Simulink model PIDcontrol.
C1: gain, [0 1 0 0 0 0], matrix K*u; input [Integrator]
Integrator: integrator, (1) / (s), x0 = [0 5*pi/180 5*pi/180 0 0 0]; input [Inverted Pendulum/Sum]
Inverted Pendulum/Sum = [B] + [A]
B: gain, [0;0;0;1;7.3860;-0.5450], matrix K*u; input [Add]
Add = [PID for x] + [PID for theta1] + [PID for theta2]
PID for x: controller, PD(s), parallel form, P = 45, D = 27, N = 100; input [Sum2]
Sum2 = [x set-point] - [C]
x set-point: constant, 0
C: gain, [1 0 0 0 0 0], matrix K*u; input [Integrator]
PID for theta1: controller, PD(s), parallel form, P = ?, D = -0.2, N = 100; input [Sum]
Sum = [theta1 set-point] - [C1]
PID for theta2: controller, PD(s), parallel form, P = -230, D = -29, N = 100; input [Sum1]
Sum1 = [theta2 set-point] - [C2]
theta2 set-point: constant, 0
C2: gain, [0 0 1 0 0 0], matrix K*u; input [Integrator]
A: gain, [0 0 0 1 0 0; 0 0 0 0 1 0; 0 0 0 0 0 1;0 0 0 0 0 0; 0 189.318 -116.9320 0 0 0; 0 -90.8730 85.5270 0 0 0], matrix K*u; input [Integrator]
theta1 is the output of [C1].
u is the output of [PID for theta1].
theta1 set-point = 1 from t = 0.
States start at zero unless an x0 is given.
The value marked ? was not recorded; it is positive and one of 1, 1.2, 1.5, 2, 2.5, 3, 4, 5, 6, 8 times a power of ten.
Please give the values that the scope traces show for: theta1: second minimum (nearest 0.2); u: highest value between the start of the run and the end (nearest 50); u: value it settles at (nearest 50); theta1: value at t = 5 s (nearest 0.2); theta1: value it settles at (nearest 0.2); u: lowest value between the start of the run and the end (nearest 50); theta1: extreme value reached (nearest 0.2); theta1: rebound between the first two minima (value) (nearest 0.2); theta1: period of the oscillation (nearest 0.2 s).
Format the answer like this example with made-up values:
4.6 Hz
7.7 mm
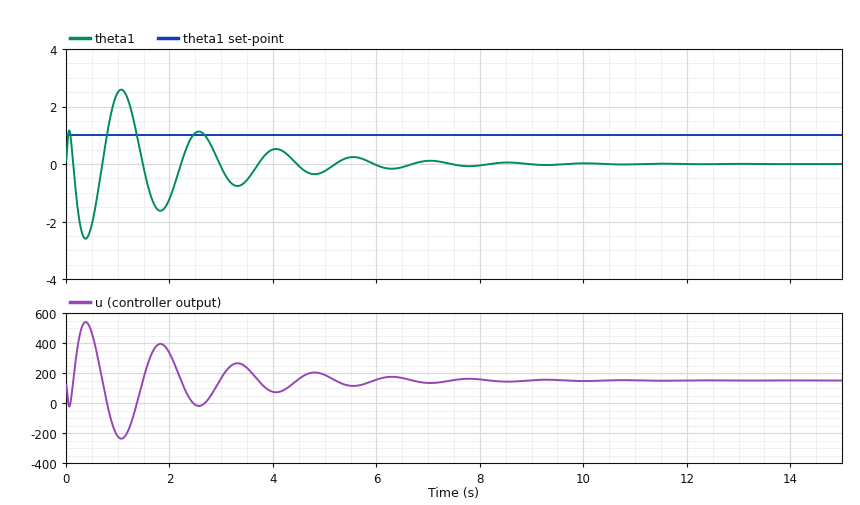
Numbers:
-1.6
550
150
-0.2
0.0
-250
-2.6
2.6
1.4 s
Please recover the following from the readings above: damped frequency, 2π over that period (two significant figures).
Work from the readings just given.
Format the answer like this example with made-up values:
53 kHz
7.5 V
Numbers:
4.5 rad/s
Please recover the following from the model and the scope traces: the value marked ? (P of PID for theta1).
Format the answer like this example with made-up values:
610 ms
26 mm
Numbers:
150
